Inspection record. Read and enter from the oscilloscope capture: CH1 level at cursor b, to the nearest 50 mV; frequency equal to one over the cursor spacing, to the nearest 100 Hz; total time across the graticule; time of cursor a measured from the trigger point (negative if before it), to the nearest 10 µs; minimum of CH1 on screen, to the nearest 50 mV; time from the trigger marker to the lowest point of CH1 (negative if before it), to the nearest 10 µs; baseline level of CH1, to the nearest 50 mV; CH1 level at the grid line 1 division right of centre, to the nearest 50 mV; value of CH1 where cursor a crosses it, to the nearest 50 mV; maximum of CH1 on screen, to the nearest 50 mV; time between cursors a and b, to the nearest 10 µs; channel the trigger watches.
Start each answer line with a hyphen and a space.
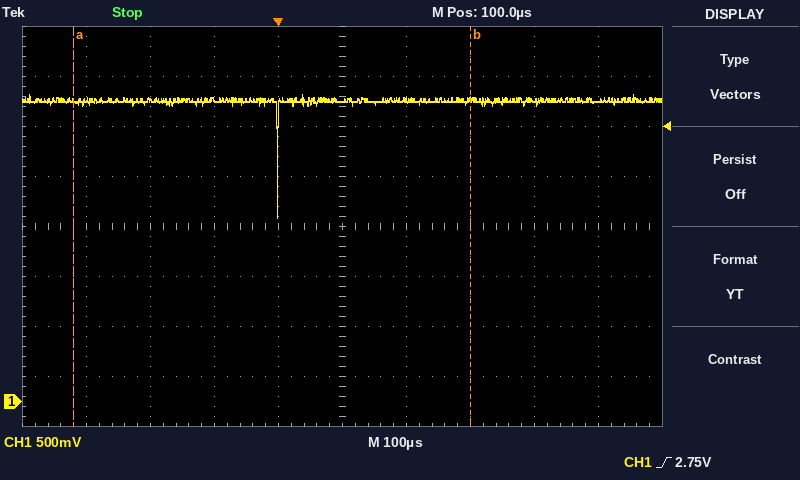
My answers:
- 3.00 V
- 1.6 kHz
- 1 ms
- -320 µs
- 1.85 V
- 0 µs
- 3.00 V
- 3.00 V
- 3.00 V
- 3.05 V
- 620 µs
- CH1
